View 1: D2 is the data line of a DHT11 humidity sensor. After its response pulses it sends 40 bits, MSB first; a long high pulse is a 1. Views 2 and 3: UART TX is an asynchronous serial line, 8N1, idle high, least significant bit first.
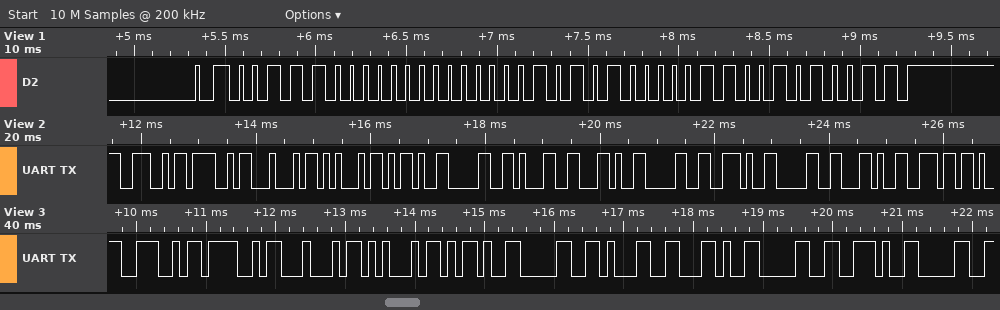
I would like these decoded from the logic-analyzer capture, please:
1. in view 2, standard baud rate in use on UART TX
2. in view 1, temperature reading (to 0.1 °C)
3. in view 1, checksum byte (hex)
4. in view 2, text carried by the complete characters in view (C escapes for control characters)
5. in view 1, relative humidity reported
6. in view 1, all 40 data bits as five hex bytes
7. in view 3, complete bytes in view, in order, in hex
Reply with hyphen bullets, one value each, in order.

- 9600 baud
- 21.6 °C
- 0x53
- "NODE-01,0.0,n"
- 56 %
- 38 00 15 06 53
- 0x4E 0x4F 0x44 0x45 0x2D 0x30 0x31 0x2C 0x30 0x2E 0x30
